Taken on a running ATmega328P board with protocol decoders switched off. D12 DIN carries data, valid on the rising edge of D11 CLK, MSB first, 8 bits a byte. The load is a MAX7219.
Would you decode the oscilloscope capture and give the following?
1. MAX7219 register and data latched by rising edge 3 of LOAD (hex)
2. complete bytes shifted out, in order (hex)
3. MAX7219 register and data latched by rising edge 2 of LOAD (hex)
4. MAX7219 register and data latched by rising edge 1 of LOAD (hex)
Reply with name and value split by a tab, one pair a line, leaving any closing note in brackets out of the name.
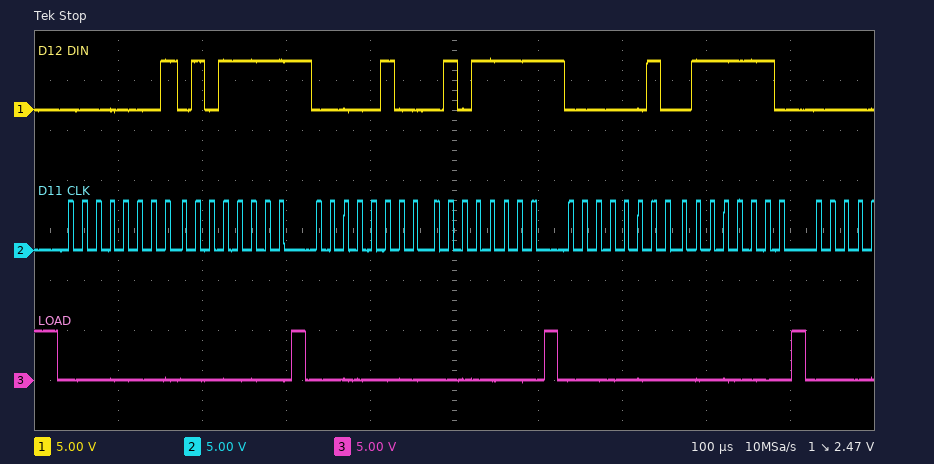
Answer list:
MAX7219 register and data latched by rising edge 3 of LOAD	register 0x2, data 0x7E
complete bytes shifted out, in order	0x01 0x5F 0x04 0x5F 0x02 0x7E
MAX7219 register and data latched by rising edge 2 of LOAD	register 0x4, data 0x5F
MAX7219 register and data latched by rising edge 1 of LOAD	register 0x1, data 0x5F
